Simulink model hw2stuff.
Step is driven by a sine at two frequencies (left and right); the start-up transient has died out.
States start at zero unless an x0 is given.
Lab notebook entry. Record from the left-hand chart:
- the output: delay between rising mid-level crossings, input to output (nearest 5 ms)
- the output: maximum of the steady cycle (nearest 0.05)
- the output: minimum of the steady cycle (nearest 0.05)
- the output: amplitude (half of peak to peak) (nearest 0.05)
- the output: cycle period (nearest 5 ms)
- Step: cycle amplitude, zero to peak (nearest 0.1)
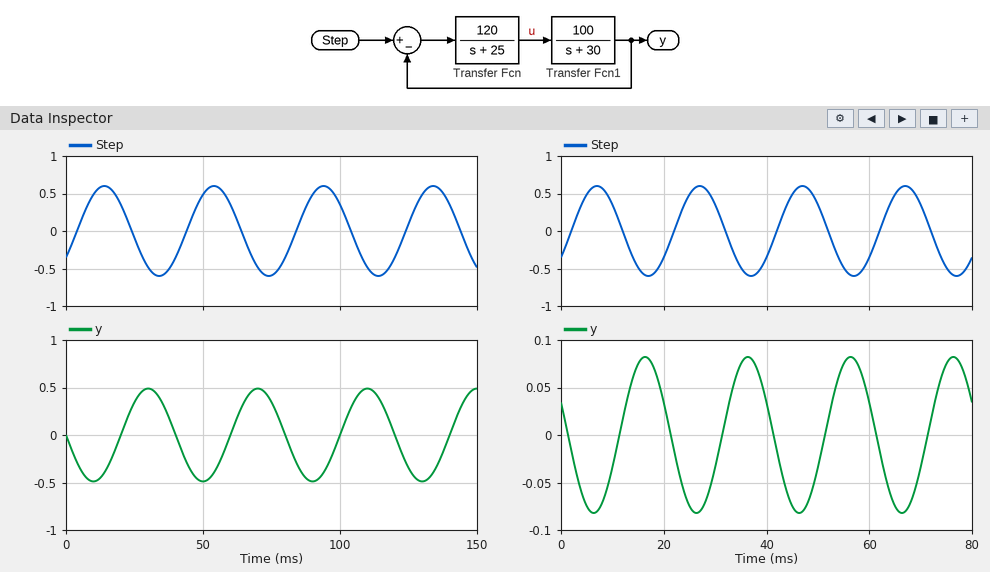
15 ms
0.50
-0.50
0.50
40 ms
0.6
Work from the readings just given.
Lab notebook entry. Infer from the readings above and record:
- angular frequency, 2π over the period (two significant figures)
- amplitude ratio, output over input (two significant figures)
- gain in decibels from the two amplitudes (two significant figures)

0.16 rad/ms
0.83
-1.6 dB
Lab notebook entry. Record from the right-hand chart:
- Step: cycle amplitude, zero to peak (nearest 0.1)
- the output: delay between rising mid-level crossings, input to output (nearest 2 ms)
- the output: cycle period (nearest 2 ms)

0.6
10 ms
20 ms
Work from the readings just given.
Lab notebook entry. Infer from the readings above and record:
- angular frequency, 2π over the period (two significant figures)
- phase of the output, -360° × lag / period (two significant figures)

0.31 rad/ms
-180°
